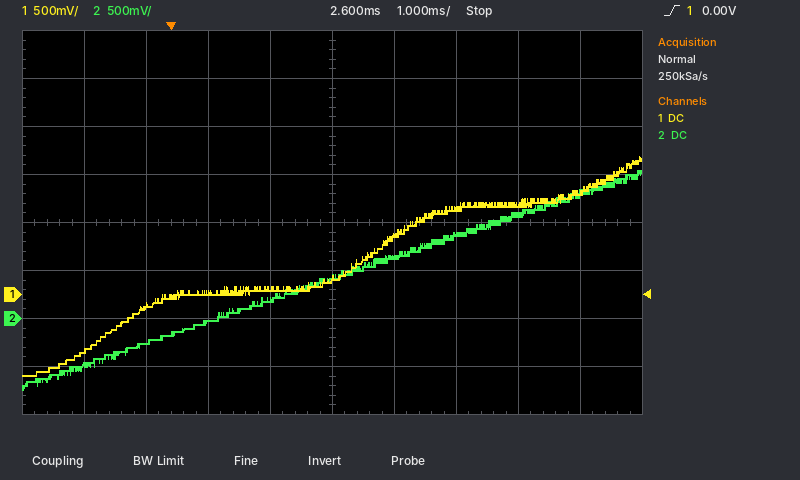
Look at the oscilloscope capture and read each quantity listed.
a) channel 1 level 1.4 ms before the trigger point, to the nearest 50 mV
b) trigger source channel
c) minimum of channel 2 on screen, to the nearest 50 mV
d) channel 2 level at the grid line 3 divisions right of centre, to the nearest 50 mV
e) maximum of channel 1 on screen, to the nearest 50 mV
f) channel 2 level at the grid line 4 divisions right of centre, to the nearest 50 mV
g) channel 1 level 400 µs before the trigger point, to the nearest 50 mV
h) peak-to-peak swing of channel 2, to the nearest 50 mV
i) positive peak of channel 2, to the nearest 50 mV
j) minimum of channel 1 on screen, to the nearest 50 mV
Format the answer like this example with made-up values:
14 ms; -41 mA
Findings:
-600 mV; channel 1; -750 mV; 1.10 V; 1.45 V; 1.30 V; -100 mV; 2.30 V; 1.55 V; -850 mV
